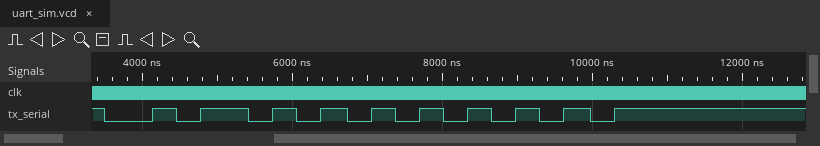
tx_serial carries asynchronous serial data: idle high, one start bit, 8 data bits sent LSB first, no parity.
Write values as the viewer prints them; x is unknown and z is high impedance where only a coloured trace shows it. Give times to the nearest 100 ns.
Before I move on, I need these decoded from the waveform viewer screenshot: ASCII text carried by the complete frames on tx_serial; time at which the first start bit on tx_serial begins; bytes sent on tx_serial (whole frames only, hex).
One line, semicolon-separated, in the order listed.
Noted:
"ZU"; 3500 ns; 5A, 55
